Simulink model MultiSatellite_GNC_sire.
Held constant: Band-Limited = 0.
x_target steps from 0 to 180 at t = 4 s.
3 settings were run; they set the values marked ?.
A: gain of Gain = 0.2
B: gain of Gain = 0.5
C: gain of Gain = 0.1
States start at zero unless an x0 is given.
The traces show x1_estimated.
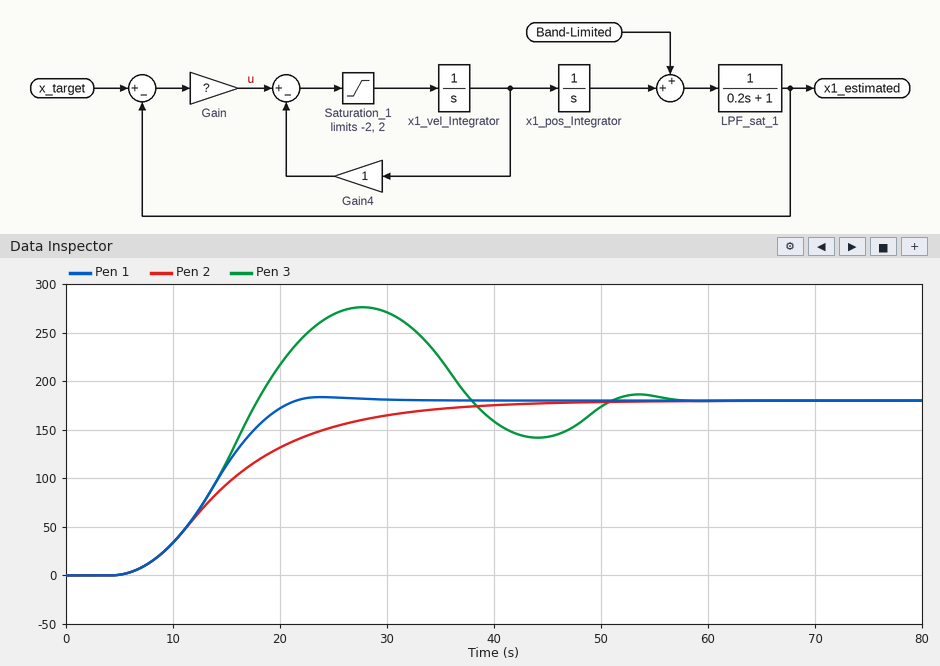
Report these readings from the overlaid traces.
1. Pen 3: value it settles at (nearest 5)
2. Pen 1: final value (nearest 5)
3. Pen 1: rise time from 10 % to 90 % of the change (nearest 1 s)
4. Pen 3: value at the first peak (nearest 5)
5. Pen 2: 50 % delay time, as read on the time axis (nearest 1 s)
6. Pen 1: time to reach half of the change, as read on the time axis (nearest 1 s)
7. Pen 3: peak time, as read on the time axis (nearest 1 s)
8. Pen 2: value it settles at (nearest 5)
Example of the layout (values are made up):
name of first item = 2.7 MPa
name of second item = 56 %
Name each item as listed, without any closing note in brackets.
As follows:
Pen 3: value it settles at = 180
Pen 1: final value = 180
Pen 1: rise time from 10 % to 90 % of the change = 10 s
Pen 3: value at the first peak = 275
Pen 2: 50 % delay time, as read on the time axis = 15 s
Pen 1: time to reach half of the change, as read on the time axis = 14 s
Pen 3: peak time, as read on the time axis = 28 s
Pen 2: value it settles at = 180
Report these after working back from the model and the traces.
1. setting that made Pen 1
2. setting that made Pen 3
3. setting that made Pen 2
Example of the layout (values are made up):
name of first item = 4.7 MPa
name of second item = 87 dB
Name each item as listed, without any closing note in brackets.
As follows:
setting that made Pen 1 = A
setting that made Pen 3 = B
setting that made Pen 2 = C
